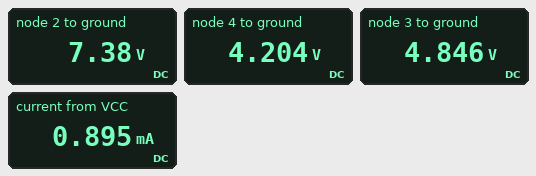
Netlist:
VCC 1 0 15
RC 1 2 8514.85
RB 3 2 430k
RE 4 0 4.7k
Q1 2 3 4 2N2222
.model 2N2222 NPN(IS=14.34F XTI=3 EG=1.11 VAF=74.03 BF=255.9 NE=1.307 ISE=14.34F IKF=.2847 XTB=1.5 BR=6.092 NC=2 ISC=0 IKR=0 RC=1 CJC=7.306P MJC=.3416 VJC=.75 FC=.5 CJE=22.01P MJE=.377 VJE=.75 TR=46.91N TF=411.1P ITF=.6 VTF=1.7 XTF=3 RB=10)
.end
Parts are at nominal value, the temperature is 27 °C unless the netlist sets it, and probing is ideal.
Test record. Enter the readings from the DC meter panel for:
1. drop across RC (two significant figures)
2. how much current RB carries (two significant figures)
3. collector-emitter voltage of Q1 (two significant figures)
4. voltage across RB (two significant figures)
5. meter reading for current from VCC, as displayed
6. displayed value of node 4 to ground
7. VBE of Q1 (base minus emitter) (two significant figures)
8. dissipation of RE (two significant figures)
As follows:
7.6 V
5.9 µA
3.2 V
2.5 V
0.895 mA
4.204 V
640 mV
3.8 mW
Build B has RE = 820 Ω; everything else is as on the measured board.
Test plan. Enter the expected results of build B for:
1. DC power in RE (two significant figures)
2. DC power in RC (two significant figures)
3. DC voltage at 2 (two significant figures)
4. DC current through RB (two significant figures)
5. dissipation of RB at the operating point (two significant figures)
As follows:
1.2 mW
12 mW
4.9 V
7.6 µA
25 µW
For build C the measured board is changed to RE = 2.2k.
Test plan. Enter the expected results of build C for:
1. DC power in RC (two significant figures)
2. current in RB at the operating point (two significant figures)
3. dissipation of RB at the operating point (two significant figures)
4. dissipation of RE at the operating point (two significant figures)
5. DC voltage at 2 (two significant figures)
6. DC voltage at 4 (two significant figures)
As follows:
9.6 mW
6.9 µA
20 µW
2.5 mW
5.9 V
2.3 V
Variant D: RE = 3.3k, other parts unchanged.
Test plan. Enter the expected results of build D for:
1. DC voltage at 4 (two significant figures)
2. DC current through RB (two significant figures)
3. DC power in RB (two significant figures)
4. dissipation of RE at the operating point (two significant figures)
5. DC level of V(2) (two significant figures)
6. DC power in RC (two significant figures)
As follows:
3.2 V
6.4 µA
18 µW
3.2 mW
6.6 V
8.2 mW
